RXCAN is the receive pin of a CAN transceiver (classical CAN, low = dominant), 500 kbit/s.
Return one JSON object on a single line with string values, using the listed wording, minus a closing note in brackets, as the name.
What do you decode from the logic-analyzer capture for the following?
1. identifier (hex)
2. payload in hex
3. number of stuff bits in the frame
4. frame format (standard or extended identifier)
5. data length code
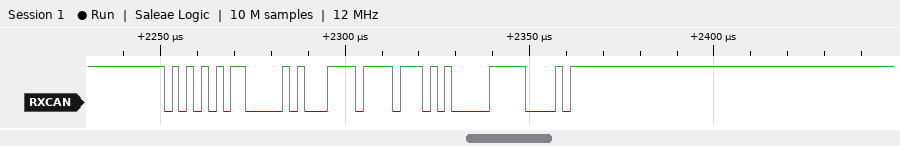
{"identifier": "0x556", "payload in hex": "3D EE", "number of stuff bits in the frame": "3", "frame format": "standard", "data length code": "2"}
